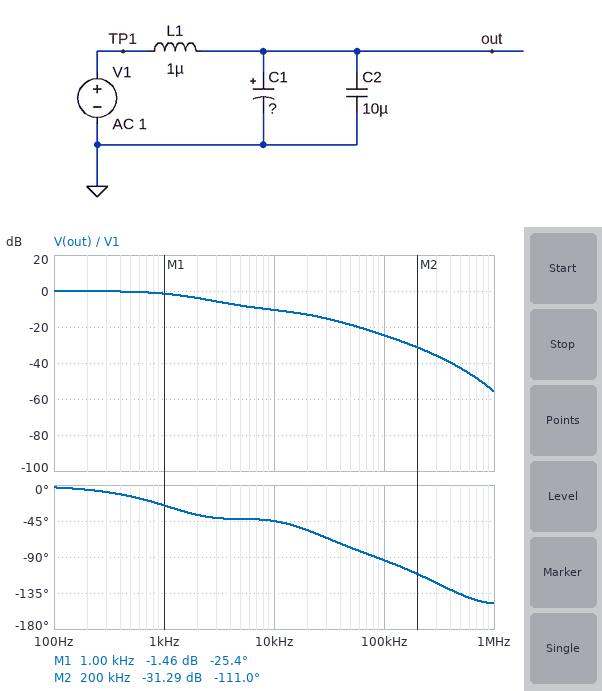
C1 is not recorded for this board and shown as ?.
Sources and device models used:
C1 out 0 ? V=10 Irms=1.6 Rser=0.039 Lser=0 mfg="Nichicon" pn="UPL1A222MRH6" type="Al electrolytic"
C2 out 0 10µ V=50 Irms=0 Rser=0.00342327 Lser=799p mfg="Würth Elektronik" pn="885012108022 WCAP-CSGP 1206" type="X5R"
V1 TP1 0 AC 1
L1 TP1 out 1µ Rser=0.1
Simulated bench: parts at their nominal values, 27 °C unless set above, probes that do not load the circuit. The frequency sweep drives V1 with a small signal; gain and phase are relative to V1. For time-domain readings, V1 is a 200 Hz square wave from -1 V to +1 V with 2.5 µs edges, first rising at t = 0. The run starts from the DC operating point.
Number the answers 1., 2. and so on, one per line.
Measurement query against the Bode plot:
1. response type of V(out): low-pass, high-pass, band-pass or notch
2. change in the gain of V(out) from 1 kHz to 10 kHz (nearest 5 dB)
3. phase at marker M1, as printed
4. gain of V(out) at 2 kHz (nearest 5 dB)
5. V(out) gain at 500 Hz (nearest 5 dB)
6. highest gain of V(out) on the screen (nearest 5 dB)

1. low-pass
2. -10 dB
3. -25.4 deg
4. -5 dB
5. 0 dB
6. 0 dB
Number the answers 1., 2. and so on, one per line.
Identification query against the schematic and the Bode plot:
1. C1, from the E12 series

1. 820 µF
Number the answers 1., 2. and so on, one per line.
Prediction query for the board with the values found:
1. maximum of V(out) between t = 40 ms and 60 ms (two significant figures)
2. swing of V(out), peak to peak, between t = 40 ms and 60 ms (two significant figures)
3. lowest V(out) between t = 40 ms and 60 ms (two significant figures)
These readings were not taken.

1. 1.0 V
2. 2.0 V
3. -1.0 V
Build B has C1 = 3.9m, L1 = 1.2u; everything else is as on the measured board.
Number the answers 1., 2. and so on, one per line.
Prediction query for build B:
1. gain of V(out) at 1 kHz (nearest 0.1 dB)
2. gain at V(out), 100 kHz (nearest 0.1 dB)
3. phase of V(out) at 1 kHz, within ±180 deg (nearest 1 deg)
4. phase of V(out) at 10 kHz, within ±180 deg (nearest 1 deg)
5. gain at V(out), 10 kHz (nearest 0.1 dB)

1. -8.1 dB
2. -26.1 dB
3. -33 deg
4. -34 deg
5. -12.0 dB
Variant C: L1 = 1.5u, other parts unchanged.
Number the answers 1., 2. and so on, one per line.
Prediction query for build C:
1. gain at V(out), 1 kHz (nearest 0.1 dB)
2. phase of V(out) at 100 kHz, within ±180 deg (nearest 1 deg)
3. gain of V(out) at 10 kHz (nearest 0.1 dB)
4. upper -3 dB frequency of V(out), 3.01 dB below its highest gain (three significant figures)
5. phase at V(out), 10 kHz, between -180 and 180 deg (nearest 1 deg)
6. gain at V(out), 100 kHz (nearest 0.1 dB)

1. -1.4 dB
2. -98 deg
3. -11.2 dB
4. 1.70 kHz
5. -56 deg
6. -28.0 dB
